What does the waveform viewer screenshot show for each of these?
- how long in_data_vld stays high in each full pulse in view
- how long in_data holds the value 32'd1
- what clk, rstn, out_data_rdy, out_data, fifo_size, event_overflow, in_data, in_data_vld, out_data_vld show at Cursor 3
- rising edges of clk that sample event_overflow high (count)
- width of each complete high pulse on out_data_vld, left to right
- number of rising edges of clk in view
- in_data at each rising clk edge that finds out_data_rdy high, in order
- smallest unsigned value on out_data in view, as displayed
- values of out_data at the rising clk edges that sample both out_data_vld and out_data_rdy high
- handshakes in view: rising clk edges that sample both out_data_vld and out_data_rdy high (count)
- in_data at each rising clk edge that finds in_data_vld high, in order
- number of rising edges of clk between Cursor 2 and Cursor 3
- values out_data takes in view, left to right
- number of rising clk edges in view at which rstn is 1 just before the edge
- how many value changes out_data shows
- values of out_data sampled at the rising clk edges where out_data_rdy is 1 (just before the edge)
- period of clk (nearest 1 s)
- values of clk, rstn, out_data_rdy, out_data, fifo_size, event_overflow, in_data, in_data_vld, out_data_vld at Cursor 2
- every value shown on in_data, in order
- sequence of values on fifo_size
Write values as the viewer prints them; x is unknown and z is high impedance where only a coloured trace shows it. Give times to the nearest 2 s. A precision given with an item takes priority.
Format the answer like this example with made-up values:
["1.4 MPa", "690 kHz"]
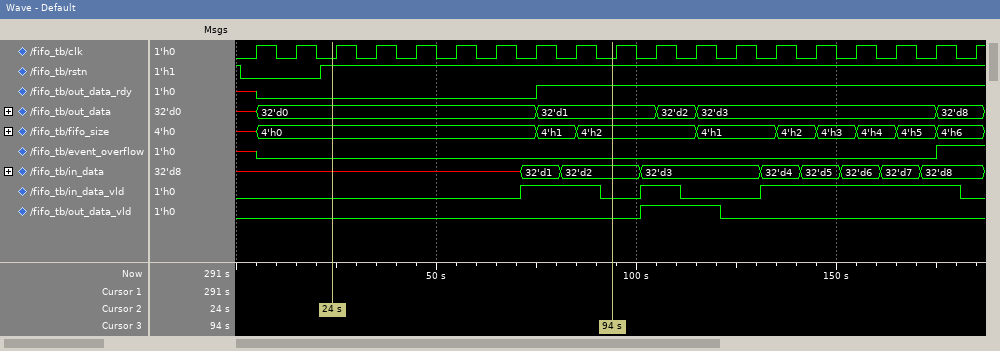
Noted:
["20 s, 10 s, 50 s", "10 s", "clk=0, rstn=1, out_data_rdy=1, out_data=32'd1, fifo_size=4'h2, event_overflow=0, in_data=32'd2, in_data_vld=0, out_data_vld=0", "1", "20 s", "19", "32'd2, 32'd2, 32'd3, 32'd3, 32'd3, 32'd4, 32'd5, 32'd6, 32'd7, 32'd8, 32'd8", "32'd0", "32'd1, 32'd2", "2", "32'd1, 32'd2, 32'd3, 32'd4, 32'd5, 32'd6, 32'd7, 32'd8", "7", "x, 32'd0, 32'd1, 32'd2, 32'd3, 32'd8", "17", "5", "32'd1, 32'd1, 32'd1, 32'd2, 32'd3, 32'd3, 32'd3, 32'd3, 32'd3, 32'd3, 32'd8", "10 s", "clk=0, rstn=1, out_data_rdy=0, out_data=32'd0, fifo_size=4'h0, event_overflow=0, in_data=x, in_data_vld=0, out_data_vld=0", "x, 32'd1, 32'd2, 32'd3, 32'd4, 32'd5, 32'd6, 32'd7, 32'd8", "x, 4'h0, 4'h1, 4'h2, 4'h1, 4'h2, 4'h3, 4'h4, 4'h5, 4'h6"]
